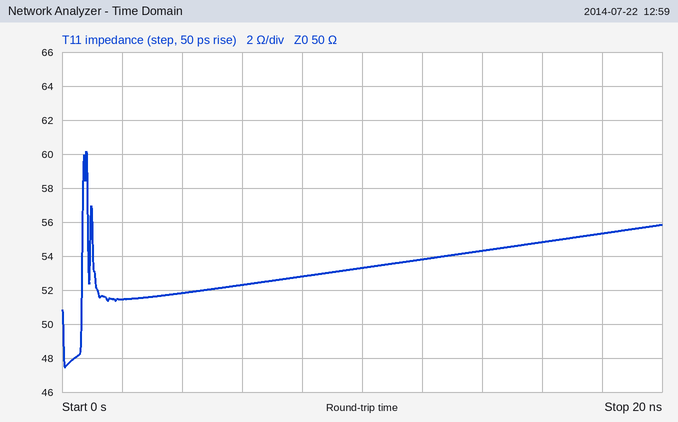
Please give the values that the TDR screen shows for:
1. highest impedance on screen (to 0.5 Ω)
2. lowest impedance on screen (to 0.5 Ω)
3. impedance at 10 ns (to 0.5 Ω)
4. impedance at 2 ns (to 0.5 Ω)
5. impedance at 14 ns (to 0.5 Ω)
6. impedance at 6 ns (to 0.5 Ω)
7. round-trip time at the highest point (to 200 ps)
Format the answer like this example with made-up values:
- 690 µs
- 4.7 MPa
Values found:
- 60.0 Ω
- 47.5 Ω
- 53.5 Ω
- 51.5 Ω
- 54.5 Ω
- 52.5 Ω
- 800 ps
